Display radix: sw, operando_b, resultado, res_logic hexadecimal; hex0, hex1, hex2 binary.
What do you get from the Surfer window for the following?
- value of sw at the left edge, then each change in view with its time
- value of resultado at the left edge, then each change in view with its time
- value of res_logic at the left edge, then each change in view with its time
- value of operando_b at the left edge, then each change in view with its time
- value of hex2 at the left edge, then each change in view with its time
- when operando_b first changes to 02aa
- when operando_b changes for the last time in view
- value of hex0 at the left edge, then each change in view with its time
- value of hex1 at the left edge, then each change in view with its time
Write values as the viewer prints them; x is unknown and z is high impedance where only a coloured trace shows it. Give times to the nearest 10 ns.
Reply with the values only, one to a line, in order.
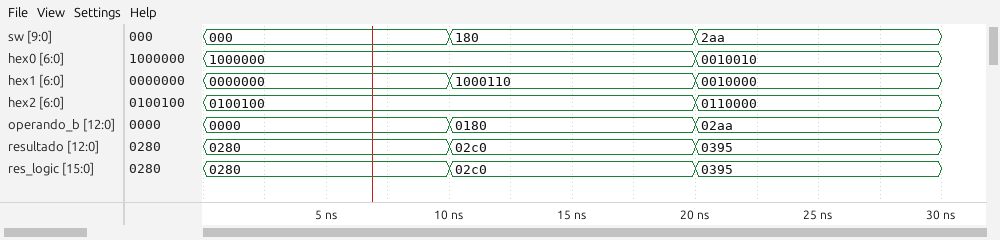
000, 180 at 10 ns, 2aa at 20 ns
0280, 02c0 at 10 ns, 0395 at 20 ns
0280, 02c0 at 10 ns, 0395 at 20 ns
0000, 0180 at 10 ns, 02aa at 20 ns
0100100, 0110000 at 20 ns
20 ns
20 ns
1000000, 0010010 at 20 ns
0000000, 1000110 at 10 ns, 0010000 at 20 ns
